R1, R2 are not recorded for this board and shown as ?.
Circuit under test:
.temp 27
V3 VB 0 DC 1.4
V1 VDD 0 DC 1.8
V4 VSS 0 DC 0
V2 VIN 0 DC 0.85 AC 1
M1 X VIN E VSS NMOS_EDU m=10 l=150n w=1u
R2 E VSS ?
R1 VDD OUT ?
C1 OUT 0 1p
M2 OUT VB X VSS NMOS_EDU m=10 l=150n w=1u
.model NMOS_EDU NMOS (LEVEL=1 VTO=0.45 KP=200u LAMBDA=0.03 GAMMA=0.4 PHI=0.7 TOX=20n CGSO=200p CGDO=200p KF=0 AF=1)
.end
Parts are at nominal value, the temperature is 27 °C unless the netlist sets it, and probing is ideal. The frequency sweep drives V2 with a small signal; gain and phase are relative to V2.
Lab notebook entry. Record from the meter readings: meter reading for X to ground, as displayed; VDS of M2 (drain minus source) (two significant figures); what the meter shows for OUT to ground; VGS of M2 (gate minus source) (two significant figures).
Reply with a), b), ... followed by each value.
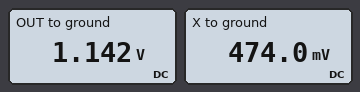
a) 474.0 mV
b) 670 mV
c) 1.142 V
d) 930 mV
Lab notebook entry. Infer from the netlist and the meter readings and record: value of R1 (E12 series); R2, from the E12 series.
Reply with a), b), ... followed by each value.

a) 680 Ω
b) 18 Ω
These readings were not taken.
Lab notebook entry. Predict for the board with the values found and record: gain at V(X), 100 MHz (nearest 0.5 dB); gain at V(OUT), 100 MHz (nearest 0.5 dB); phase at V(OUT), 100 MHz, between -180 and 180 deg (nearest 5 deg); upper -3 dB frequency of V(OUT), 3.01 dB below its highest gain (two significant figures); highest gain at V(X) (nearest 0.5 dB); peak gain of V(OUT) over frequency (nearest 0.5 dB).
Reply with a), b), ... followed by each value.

a) -2.5 dB
b) 9.0 dB
c) 155 deg
d) 230 MHz
e) -2.5 dB
f) 10.0 dB
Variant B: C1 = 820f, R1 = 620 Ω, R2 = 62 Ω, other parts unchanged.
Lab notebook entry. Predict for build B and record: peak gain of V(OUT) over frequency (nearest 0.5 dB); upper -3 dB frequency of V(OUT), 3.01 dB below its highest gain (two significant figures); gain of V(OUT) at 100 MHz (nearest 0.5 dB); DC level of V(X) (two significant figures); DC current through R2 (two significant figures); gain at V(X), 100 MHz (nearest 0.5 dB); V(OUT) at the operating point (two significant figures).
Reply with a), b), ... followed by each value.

a) 6.5 dB
b) 310 MHz
c) 6.0 dB
d) 510 mV
e) 780 µA
f) -4.0 dB
g) 1.3 V
